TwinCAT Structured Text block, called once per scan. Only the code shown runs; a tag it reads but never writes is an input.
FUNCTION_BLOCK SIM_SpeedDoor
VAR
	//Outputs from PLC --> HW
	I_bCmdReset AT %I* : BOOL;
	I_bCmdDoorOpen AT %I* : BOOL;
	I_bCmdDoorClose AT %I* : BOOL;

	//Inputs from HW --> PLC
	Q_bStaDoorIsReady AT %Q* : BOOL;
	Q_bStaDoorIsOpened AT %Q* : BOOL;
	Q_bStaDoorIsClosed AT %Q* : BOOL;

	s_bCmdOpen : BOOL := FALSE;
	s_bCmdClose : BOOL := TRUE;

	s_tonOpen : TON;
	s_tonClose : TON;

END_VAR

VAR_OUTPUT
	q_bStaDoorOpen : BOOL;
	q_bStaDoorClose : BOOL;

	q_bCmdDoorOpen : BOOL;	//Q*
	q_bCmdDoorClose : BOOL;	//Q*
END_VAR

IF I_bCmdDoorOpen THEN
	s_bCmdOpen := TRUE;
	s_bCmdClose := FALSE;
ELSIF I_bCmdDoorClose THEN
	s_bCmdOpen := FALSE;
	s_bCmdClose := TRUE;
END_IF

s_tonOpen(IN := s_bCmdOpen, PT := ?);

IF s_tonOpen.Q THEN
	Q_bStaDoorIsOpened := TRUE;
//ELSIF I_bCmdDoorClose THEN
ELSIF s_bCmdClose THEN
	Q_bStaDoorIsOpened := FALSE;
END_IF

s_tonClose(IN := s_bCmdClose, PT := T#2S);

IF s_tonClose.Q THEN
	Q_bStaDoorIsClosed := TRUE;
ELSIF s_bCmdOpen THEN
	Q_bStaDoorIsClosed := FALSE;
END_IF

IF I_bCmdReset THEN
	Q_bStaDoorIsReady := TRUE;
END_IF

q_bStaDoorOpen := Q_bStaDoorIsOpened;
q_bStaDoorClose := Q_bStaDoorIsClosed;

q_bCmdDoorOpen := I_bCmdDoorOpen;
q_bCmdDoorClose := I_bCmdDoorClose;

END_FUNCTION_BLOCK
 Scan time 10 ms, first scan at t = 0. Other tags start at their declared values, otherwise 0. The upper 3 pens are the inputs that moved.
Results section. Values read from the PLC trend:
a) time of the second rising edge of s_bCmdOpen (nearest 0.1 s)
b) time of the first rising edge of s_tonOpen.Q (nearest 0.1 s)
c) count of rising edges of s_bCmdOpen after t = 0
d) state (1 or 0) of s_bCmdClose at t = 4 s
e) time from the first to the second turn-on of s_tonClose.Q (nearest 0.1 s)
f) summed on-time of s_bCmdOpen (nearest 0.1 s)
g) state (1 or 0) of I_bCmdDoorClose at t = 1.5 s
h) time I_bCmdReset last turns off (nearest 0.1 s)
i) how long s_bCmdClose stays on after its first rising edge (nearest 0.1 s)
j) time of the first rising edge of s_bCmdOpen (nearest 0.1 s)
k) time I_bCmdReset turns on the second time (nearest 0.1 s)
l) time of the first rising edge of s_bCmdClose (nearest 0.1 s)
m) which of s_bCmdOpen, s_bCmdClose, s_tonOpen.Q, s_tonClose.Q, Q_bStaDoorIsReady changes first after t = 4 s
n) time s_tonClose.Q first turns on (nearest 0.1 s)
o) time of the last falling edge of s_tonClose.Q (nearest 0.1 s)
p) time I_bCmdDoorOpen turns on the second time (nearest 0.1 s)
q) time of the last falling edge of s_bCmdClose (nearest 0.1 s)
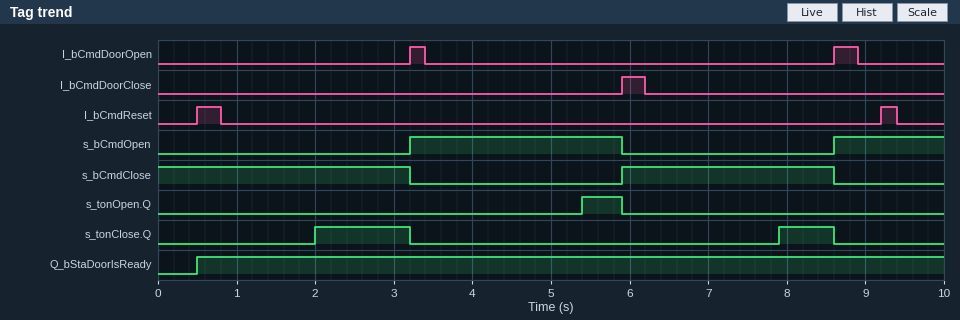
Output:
8.6 s
5.4 s
2
0
5.9 s
4.1 s
0
9.4 s
2.7 s
3.2 s
9.2 s
5.9 s
s_tonOpen.Q
2.0 s
8.6 s
8.6 s
8.6 s
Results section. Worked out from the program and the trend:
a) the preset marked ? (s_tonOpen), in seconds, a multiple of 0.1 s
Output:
2.2 s
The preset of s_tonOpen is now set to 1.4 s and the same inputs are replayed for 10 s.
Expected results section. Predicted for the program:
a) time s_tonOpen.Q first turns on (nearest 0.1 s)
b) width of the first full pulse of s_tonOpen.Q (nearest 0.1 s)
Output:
4.6 s
1.3 s
